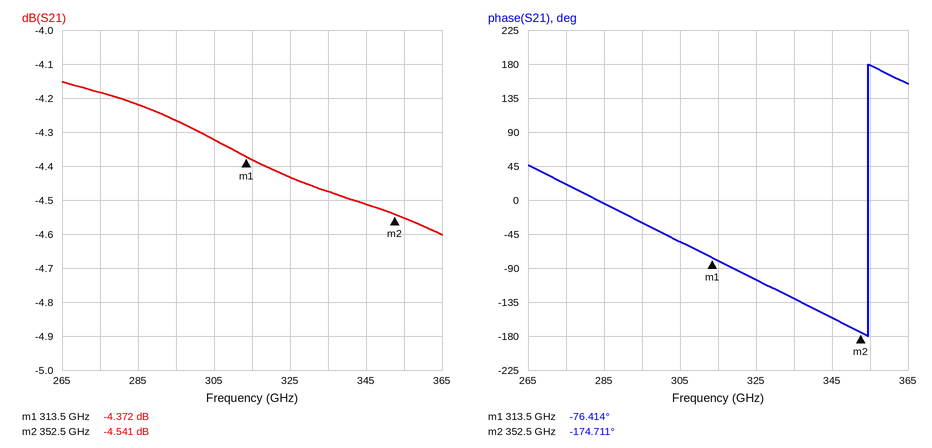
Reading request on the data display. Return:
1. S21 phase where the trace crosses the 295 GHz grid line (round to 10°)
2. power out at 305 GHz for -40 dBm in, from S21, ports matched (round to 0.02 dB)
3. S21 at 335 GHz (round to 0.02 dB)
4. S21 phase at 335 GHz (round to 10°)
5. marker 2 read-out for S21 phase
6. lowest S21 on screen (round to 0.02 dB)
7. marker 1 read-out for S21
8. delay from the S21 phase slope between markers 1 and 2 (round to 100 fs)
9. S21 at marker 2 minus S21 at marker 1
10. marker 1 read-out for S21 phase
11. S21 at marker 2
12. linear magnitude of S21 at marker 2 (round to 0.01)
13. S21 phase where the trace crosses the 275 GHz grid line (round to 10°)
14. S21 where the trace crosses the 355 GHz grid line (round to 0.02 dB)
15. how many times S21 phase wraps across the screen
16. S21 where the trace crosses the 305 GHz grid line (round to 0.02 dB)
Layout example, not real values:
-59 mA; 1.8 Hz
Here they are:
-30°; -44.32 dBm; -4.48 dB; -130°; -174.711°; -4.60 dB; -4.372 dB; 7.0 ps; -0.169 dB; -76.414°; -4.541 dB; 0.59; 20°; -4.56 dB; 1; -4.32 dB
